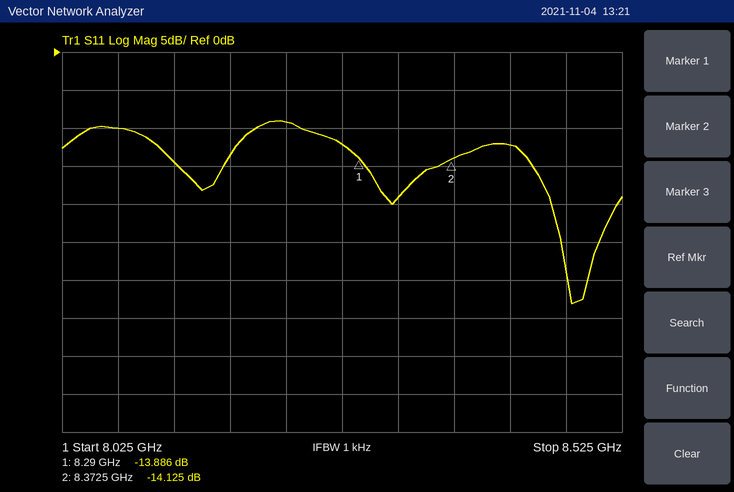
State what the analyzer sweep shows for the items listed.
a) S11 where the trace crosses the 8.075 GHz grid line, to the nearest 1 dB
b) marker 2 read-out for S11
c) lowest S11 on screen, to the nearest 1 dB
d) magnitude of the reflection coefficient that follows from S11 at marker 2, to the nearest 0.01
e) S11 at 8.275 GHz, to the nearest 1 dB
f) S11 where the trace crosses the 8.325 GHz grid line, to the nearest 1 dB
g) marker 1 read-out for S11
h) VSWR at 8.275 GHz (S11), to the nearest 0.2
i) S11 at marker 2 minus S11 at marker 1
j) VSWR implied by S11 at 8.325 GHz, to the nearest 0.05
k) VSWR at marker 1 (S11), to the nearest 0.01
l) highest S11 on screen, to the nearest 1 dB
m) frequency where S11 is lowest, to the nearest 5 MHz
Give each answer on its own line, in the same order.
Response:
-10 dB
-14.125 dB
-33 dB
0.20
-12 dB
-19 dB
-13.886 dB
1.6
-0.239 dB
1.25
1.51
-9 dB
8.480 GHz
